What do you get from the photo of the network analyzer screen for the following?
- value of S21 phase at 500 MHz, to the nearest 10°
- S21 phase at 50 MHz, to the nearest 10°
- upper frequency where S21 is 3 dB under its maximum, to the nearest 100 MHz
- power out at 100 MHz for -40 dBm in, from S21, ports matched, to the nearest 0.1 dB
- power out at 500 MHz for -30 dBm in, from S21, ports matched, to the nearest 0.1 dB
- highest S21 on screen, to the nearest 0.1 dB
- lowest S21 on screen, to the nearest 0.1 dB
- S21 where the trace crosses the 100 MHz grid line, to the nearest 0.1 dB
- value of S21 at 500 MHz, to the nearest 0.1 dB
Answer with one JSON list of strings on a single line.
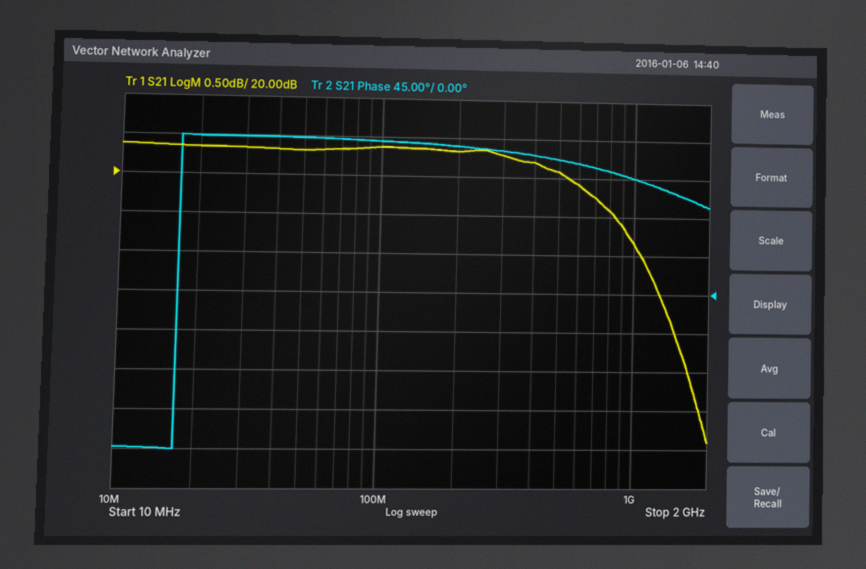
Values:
["160°", "180°", "1.7 GHz", "-19.6 dBm", "-9.9 dBm", "20.4 dB", "16.6 dB", "20.4 dB", "20.1 dB"]
